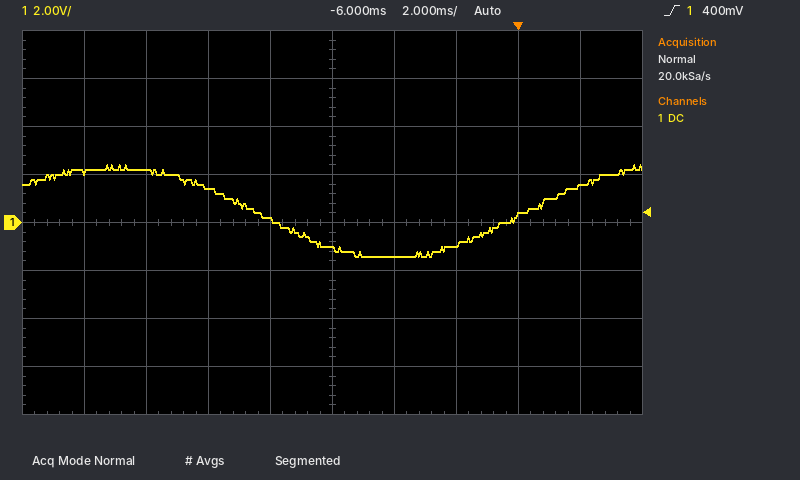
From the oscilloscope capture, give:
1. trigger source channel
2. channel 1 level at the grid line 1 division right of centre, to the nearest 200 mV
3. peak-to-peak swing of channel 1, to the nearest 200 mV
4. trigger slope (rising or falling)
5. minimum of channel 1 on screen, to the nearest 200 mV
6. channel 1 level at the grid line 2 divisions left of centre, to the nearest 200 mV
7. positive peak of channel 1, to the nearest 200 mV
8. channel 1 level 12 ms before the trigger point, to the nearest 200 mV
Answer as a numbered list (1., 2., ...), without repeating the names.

1. channel 1
2. -1.4 V
3. 3.8 V
4. rising
5. -1.4 V
6. 1.4 V
7. 2.4 V
8. 2.2 V
